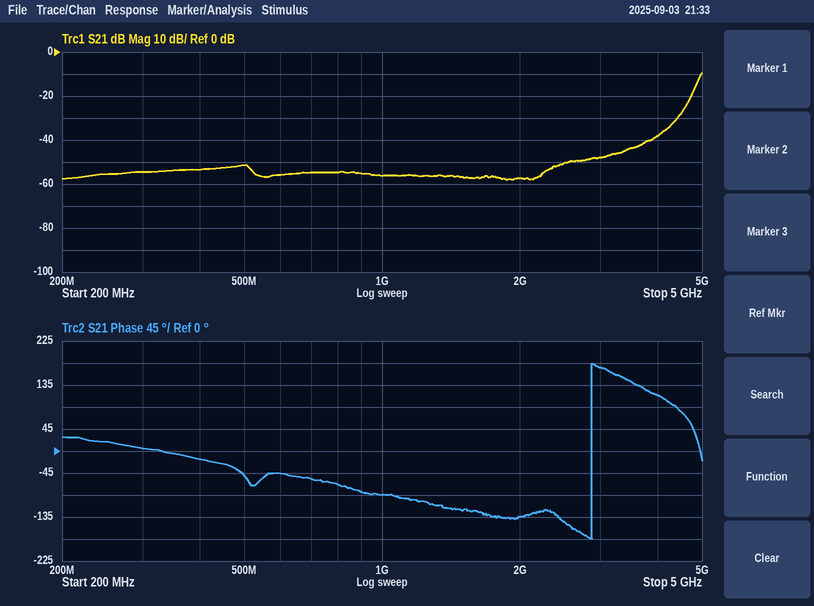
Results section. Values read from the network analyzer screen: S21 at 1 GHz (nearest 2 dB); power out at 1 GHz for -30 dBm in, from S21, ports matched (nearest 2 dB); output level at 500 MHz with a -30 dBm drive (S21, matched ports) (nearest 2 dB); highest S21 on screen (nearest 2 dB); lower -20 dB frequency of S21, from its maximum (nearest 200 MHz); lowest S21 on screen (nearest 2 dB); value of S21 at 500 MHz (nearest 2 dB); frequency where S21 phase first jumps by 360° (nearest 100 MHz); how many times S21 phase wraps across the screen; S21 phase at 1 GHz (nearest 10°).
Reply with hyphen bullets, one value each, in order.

- -56 dB
- -86 dBm
- -82 dBm
- -10 dB
- 4.4 GHz
- -58 dB
- -52 dB
- 2.9 GHz
- 1
- -90°
